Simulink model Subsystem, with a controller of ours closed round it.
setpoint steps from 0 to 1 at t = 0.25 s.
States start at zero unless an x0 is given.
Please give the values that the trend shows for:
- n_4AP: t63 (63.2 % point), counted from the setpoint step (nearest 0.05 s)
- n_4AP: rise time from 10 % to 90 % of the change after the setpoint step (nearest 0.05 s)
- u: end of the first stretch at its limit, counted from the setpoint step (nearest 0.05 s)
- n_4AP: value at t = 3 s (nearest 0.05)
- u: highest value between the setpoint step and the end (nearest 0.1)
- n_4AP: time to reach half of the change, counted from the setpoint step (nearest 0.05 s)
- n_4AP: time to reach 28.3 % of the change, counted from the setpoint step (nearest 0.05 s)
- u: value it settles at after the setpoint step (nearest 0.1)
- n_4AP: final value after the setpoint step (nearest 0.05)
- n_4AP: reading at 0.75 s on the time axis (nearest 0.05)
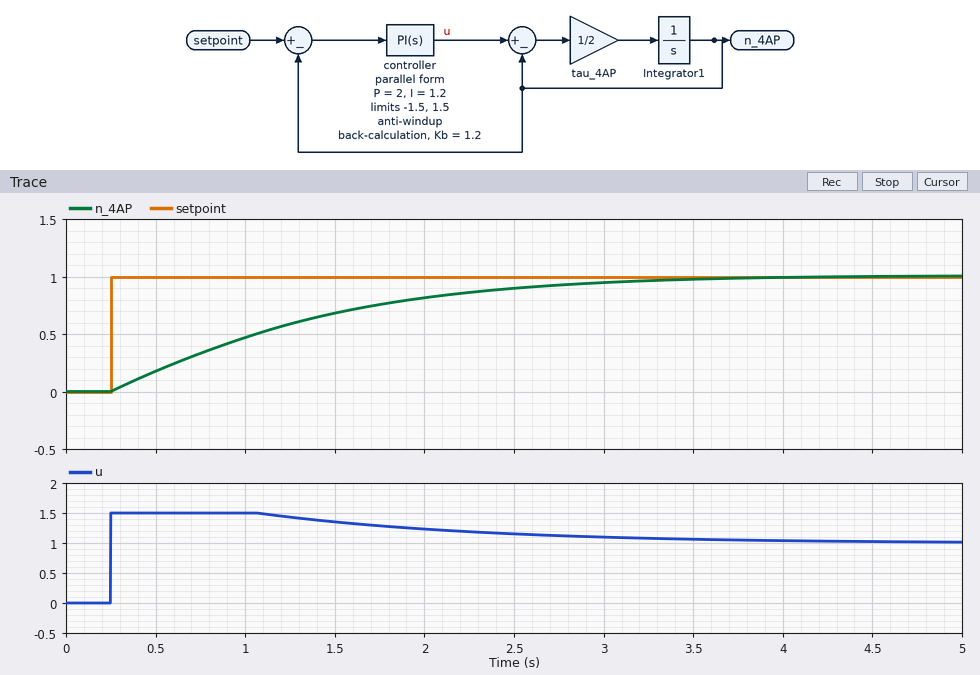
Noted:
1.10 s
2.15 s
0.85 s
0.95
1.5
0.80 s
0.40 s
1.0
1.00
0.35
